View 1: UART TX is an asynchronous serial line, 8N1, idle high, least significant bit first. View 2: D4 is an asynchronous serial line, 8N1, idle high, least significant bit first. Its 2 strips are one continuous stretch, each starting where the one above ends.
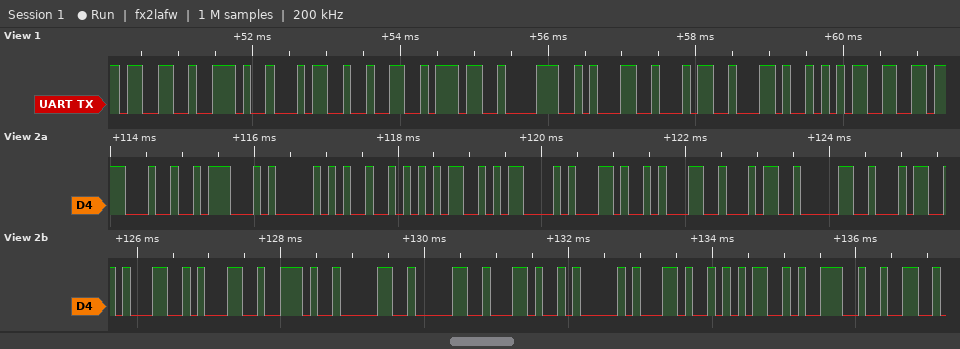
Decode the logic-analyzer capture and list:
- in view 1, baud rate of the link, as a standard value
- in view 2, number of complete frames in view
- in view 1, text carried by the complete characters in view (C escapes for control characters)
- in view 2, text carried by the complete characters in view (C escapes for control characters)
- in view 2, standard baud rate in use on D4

9600 baud
22
"3.427814,5"
"$GPRMC,140411.00,A,592"
9600 baud
